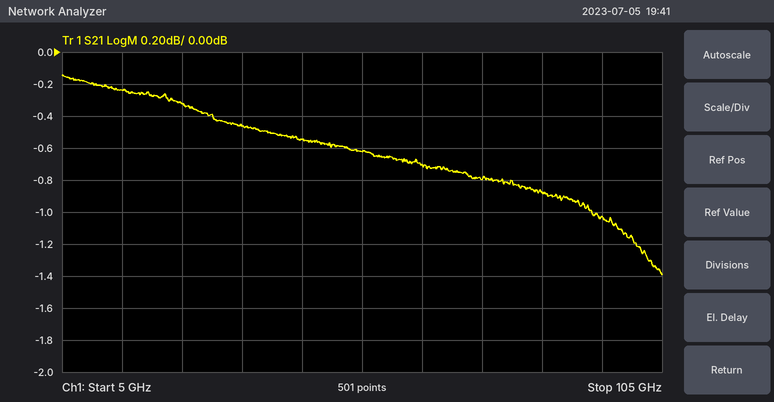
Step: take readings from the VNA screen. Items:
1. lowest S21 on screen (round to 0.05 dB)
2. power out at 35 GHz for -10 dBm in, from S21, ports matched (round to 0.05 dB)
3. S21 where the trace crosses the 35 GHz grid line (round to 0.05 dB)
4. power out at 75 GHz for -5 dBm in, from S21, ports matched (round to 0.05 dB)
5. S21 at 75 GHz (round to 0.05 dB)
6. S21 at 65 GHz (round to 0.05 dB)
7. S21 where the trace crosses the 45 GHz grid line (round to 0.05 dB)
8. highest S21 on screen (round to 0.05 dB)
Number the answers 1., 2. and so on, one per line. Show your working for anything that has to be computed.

1. -1.40 dB
2. -10 dBm + (-0.45 dB) = -10.45 dBm
3. -0.45 dB
4. -5 dBm + (-0.80 dB) = -5.80 dBm
5. -0.80 dB
6. -0.70 dB
7. -0.55 dB
8. -0.15 dB
